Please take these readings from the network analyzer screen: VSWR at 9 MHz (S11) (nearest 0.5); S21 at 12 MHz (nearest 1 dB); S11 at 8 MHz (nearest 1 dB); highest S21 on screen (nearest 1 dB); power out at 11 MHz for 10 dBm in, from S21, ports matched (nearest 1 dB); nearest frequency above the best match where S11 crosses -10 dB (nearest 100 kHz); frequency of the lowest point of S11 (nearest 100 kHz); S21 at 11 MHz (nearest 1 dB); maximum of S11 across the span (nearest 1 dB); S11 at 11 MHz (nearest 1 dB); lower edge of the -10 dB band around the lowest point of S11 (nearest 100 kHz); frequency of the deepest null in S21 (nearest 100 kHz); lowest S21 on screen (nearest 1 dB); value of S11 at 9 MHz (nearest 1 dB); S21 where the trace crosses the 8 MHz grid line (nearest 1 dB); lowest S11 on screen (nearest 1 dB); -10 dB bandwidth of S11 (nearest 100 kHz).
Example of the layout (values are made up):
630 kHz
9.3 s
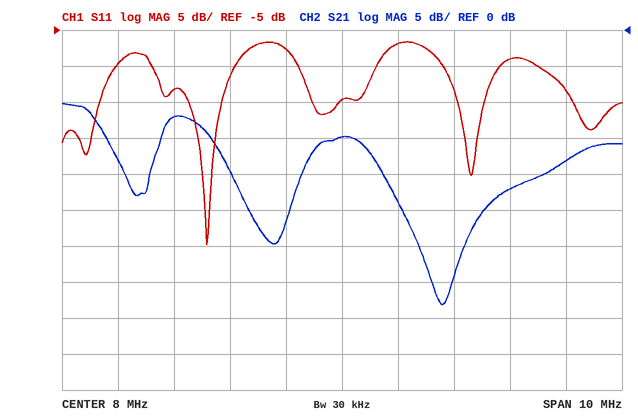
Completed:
2.5
-18 dB
-15 dB
-10 dB
-12 dBm
6.1 MHz
5.6 MHz
-22 dB
-7 dB
-9 dB
4.6 MHz
9.8 MHz
-38 dB
-7 dB
-15 dB
-35 dB
1.5 MHz
